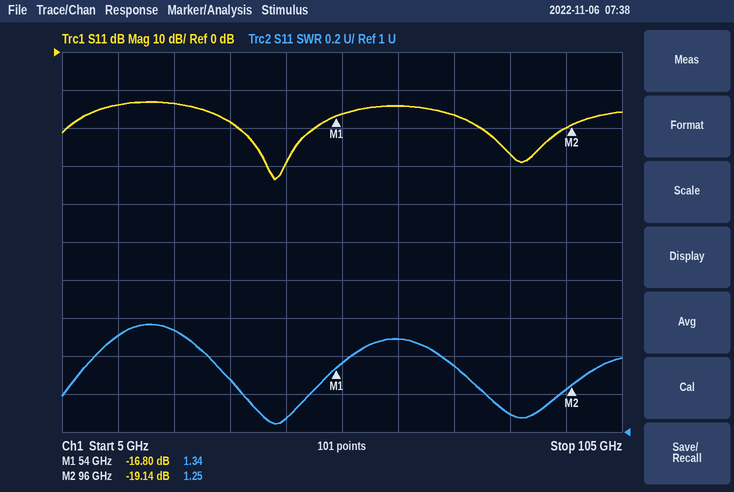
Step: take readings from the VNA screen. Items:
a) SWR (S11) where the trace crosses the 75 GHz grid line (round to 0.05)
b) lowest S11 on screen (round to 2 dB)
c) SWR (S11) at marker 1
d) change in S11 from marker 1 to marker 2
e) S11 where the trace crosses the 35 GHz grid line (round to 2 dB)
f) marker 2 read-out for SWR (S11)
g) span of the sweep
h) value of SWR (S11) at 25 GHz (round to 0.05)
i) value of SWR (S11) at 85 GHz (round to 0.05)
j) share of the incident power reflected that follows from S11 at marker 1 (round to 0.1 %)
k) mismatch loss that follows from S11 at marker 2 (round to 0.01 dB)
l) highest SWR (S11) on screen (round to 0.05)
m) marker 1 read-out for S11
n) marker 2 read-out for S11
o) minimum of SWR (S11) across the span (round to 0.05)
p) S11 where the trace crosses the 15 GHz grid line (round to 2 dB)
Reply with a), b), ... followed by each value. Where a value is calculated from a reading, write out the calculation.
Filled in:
a) 1.35
b) -34 dB
c) 1.34
d) -19.14 − (-16.8) = -2.34 dB
e) -18 dB
f) 1.25
g) 100 GHz
h) 1.55
i) 1.10
j) 10^(-16.8/10) ≈ 2.1 %
k) −10 log10(1 − 10^(-19.14/10)) ≈ 0.05 dB
l) 1.55
m) -16.80 dB
n) -19.14 dB
o) 1.05
p) -14 dB
